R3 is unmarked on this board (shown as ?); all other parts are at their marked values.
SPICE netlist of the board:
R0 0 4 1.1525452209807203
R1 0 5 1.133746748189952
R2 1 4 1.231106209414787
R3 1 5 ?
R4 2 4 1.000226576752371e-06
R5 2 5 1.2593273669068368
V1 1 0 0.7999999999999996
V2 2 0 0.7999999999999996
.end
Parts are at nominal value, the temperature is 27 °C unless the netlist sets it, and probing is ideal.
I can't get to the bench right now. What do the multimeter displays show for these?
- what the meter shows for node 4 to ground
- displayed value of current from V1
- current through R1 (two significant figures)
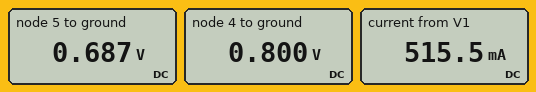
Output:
0.800 V
515.5 mA
610 mA
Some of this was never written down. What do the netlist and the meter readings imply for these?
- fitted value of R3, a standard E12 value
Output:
0.22 Ω
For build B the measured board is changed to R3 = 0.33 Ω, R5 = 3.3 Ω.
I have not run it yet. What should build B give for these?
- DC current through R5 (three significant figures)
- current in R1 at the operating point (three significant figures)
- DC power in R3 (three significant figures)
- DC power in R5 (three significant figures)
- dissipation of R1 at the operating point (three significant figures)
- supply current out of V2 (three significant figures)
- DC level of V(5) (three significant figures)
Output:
50.7 mA
558 mA
84.9 mW
8.49 mW
353 mW
745 mA
633 mV
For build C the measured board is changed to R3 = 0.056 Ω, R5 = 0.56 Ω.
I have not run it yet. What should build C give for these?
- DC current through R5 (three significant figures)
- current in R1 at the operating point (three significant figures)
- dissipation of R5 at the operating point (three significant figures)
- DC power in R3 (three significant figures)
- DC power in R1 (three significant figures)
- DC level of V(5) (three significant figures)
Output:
61.4 mA
675 mA
2.11 mW
21.1 mW
517 mW
766 mV
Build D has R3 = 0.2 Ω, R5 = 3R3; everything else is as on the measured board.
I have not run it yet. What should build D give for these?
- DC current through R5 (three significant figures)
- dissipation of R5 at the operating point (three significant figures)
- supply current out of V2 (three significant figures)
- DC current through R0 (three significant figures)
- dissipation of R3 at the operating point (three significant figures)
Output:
34.6 mA
3.94 mW
729 mA
694 mA
65.1 mW
